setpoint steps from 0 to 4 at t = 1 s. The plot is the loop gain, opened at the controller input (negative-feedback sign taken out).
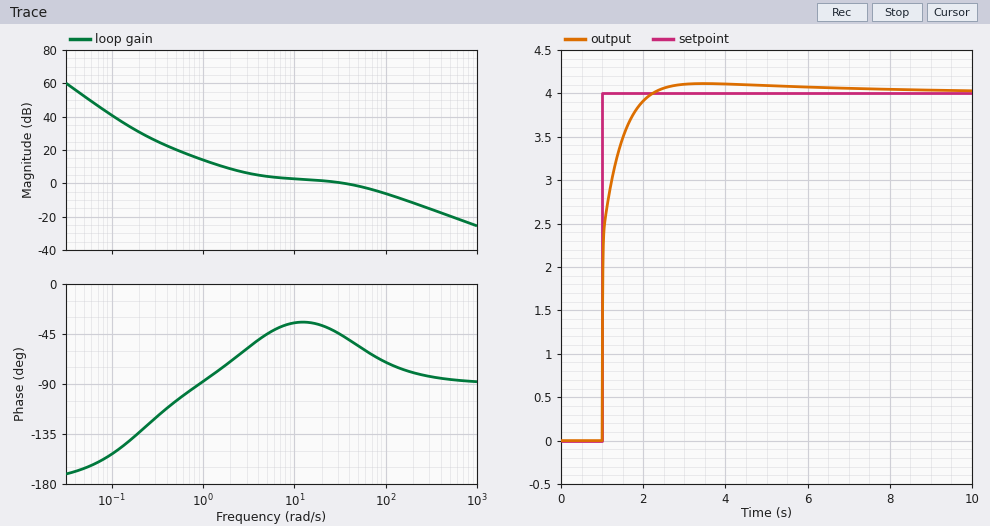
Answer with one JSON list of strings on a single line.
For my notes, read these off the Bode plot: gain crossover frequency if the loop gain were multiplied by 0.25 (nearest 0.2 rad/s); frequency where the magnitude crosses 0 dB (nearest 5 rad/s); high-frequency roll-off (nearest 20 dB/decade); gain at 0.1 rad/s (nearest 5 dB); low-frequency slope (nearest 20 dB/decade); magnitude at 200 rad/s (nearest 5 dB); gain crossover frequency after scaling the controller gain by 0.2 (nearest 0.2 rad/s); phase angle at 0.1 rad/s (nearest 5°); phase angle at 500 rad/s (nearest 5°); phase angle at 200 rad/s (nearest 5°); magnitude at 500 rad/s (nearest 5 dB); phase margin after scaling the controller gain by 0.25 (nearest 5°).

["1.2 rad/s", "35 rad/s", "-20 dB/decade", "40 dB", "-40 dB/decade", "-10 dB", "1.0 rad/s", "-155°", "-85°", "-80°", "-20 dB", "100°"]
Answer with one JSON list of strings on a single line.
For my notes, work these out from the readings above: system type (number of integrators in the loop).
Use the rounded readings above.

["2"]
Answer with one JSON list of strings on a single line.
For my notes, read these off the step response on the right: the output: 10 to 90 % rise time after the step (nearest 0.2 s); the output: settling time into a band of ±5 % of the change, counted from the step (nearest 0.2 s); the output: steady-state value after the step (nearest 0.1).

["0.6 s", "0.8 s", "4.0"]
